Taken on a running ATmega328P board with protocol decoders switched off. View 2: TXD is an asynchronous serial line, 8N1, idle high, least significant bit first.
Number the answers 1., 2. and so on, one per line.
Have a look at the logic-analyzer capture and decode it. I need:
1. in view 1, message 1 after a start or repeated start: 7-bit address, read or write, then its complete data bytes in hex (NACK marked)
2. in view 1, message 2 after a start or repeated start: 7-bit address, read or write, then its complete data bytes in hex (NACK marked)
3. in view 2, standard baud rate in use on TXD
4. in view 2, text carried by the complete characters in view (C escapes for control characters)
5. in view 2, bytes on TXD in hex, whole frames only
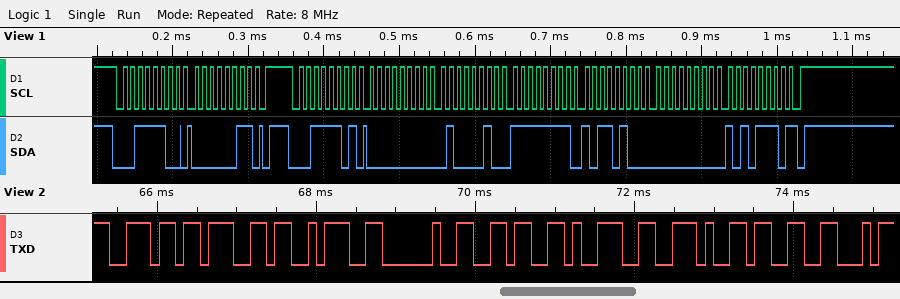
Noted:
1. 0x1E write: 03
2. 0x1E read: 00 42 FF B4 00 AE NACK
3. 9600 baud
4. "ng: 69.3"
5. 6E 67 3A 20 36 39 2E 33
